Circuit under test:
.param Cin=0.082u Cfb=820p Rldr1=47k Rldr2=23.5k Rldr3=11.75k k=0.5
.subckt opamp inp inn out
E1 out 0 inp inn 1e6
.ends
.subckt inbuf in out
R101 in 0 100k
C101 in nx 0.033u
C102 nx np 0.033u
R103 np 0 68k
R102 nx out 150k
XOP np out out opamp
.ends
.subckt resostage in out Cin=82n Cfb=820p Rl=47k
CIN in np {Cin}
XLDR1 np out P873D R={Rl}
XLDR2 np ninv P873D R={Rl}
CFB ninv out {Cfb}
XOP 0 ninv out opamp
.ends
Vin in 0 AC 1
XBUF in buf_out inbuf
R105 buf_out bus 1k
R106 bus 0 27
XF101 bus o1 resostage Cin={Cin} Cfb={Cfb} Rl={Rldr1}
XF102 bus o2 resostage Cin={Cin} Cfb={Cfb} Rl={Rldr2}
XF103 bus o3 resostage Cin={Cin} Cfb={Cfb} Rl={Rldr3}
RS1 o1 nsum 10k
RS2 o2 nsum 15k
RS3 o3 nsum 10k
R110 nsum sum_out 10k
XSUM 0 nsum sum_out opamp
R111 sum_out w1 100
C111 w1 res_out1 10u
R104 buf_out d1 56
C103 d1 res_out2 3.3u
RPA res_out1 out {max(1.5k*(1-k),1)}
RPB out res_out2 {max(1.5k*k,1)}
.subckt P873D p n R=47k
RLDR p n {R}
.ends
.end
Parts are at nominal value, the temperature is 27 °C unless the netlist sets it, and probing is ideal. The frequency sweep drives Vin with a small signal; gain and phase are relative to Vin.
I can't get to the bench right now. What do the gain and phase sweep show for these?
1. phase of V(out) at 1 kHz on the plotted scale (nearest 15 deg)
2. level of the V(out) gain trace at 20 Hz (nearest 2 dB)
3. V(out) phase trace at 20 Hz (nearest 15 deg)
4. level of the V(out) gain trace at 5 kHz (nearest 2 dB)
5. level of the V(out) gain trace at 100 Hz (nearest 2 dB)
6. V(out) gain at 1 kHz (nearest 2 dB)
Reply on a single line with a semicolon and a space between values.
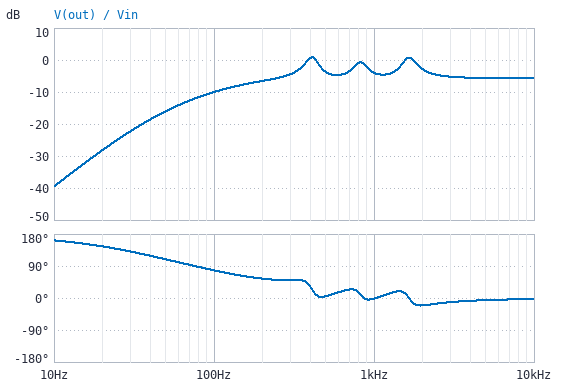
0 deg; -28 dB; 150 deg; -6 dB; -10 dB; -4 dB
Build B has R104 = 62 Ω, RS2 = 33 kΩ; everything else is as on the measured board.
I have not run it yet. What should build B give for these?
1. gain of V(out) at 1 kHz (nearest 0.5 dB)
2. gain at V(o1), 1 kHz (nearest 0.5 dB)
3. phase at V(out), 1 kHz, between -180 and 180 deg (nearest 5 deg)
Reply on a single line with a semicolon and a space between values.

-5.0 dB; -18.0 dB; 5 deg
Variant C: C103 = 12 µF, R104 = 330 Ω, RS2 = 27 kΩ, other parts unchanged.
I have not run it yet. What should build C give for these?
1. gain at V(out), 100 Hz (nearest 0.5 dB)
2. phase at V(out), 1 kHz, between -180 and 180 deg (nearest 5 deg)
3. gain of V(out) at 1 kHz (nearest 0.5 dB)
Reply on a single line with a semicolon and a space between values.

-11.0 dB; 5 deg; -5.5 dB
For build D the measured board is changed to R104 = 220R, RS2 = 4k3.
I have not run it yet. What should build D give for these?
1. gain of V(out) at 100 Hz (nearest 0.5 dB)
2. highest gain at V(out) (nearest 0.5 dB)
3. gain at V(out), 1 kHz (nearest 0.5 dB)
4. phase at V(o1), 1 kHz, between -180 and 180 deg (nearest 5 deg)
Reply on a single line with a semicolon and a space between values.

-10.5 dB; 6.0 dB; 0 dB; 105 deg
